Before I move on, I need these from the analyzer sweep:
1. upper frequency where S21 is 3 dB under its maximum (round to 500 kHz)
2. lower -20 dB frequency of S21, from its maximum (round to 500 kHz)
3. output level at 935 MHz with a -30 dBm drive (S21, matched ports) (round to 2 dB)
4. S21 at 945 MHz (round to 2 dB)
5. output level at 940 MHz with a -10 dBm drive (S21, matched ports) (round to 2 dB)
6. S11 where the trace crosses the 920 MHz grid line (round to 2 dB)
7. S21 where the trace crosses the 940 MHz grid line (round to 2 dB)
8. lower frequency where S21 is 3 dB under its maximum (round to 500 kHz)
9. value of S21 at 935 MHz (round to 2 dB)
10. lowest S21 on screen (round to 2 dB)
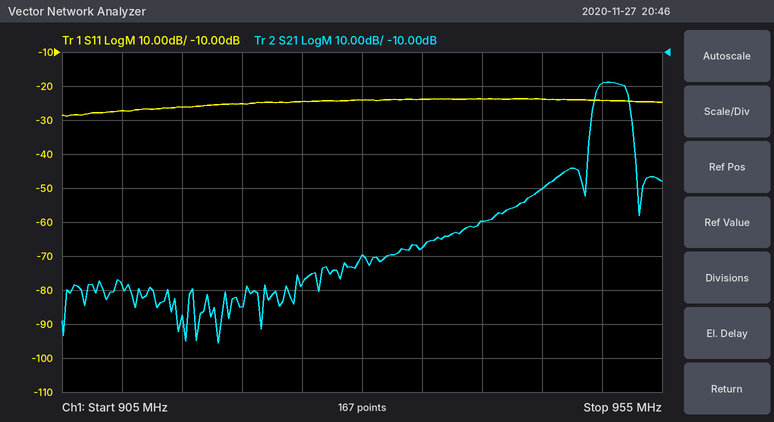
952.0 MHz
949.0 MHz
-98 dBm
-50 dB
-70 dBm
-26 dB
-60 dB
949.5 MHz
-68 dB
-96 dB
